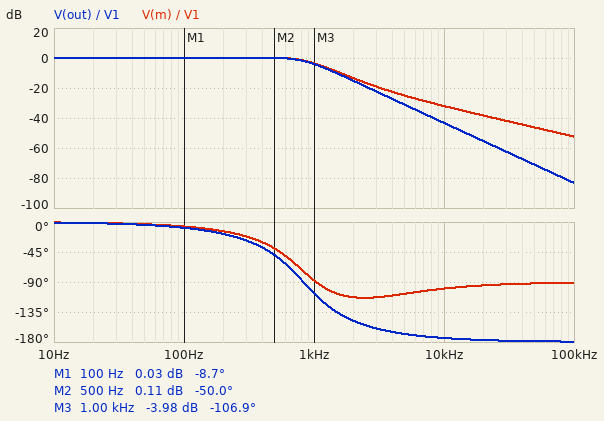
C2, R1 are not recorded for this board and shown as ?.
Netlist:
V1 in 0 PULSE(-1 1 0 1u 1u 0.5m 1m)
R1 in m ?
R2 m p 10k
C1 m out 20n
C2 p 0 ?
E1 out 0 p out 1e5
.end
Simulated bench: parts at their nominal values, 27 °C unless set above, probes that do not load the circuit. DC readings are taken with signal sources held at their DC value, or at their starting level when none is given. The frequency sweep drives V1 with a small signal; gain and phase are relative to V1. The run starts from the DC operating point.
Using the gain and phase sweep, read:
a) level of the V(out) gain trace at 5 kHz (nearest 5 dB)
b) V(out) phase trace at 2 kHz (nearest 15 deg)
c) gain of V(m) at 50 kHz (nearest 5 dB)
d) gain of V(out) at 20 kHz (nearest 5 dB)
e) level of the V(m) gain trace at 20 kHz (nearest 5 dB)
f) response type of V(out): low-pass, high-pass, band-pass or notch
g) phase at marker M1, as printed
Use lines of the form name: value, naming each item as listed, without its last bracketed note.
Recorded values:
level of the V(out) gain trace at 5 kHz: -30 dB
V(out) phase trace at 2 kHz: -150 deg
gain of V(m) at 50 kHz: -45 dB
gain of V(out) at 20 kHz: -55 dB
level of the V(m) gain trace at 20 kHz: -40 dB
response type of V(out): low-pass, high-pass, band-pass or notch: low-pass
phase at marker M1, as printed: -8.7 deg
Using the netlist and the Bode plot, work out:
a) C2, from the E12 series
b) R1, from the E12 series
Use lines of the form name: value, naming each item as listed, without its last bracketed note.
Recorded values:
C2, from the E12 series: 5.6 nF
R1, from the E12 series: 33 kΩ
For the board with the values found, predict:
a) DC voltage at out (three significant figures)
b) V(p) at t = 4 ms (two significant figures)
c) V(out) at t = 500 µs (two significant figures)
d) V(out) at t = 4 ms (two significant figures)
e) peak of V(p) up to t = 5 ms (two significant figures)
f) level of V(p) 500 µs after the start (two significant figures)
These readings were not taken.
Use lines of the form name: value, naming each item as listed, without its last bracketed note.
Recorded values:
DC voltage at out: -1.00 V
V(p) at t = 4 ms: -780 mV
V(out) at t = 500 µs: 890 mV
V(out) at t = 4 ms: -780 mV
peak of V(p) up to t = 5 ms: 940 mV
level of V(p) 500 µs after the start: 890 mV
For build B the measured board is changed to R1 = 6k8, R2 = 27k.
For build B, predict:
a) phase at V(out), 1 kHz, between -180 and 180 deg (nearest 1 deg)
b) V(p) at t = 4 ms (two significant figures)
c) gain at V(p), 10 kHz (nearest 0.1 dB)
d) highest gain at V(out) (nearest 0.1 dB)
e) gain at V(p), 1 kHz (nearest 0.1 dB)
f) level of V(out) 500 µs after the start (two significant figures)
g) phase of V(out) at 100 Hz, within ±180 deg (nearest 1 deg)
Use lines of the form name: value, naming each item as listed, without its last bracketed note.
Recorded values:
phase at V(out), 1 kHz, between -180 and 180 deg: -81 deg
V(p) at t = 4 ms: -1.1 V
gain at V(p), 10 kHz: -38.2 dB
highest gain at V(out): 0.1 dB
gain at V(p), 1 kHz: -1.6 dB
level of V(out) 500 µs after the start: 1.1 V
phase of V(out) at 100 Hz, within ±180 deg: -7 deg
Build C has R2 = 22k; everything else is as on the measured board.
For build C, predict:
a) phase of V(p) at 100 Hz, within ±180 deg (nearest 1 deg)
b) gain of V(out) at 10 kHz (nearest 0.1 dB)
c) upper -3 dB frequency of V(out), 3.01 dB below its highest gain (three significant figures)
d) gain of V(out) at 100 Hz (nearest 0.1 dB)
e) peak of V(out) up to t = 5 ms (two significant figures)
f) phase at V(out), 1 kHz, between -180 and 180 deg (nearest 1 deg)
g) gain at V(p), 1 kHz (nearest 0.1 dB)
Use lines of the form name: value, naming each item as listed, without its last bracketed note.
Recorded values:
phase of V(p) at 100 Hz, within ±180 deg: -11 deg
gain of V(out) at 10 kHz: -50.1 dB
upper -3 dB frequency of V(out), 3.01 dB below its highest gain: 643 Hz
gain of V(out) at 100 Hz: 0.1 dB
peak of V(out) up to t = 5 ms: 630 mV
phase at V(out), 1 kHz, between -180 and 180 deg: -139 deg
gain at V(p), 1 kHz: -9.4 dB
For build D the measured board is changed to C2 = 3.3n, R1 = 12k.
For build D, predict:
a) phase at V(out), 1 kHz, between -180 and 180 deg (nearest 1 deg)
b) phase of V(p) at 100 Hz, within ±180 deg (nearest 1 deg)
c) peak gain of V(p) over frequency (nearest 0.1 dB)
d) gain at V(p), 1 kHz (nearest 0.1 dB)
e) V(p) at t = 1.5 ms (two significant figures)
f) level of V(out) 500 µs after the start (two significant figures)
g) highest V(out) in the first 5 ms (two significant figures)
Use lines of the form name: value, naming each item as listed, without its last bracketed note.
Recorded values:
phase at V(out), 1 kHz, between -180 and 180 deg: -34 deg
phase of V(p) at 100 Hz, within ±180 deg: -3 deg
peak gain of V(p) over frequency: 2.6 dB
gain at V(p), 1 kHz: 1.7 dB
V(p) at t = 1.5 ms: 980 mV
level of V(out) 500 µs after the start: 1.0 V
highest V(out) in the first 5 ms: 1.5 V
